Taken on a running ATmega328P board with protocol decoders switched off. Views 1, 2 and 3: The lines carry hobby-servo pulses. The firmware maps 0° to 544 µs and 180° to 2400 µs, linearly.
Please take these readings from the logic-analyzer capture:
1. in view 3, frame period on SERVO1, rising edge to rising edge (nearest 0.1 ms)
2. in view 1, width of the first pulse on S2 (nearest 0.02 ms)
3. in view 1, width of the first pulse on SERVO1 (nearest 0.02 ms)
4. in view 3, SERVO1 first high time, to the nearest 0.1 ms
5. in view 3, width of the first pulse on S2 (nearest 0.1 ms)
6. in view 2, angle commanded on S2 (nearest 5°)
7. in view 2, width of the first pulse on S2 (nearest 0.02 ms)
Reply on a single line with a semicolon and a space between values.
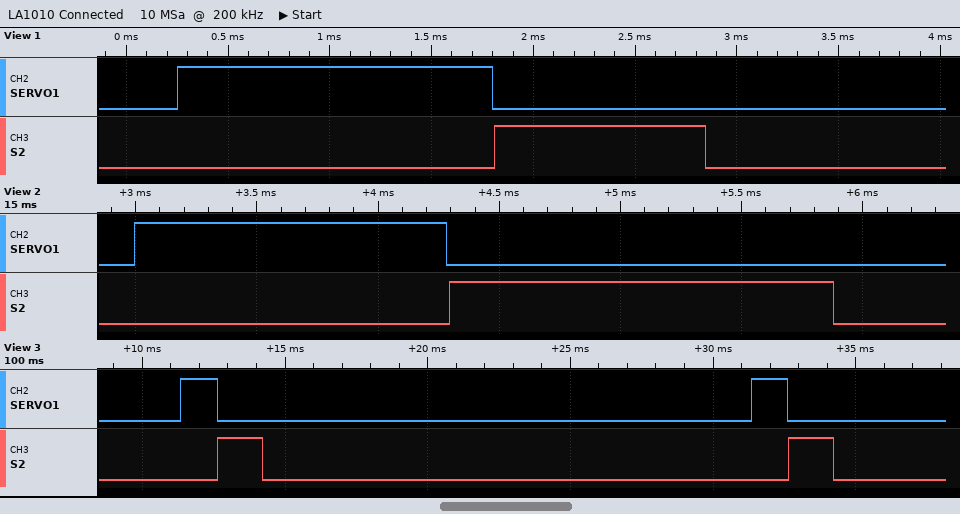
20.0 ms; 1.04 ms; 1.54 ms; 1.3 ms; 1.6 ms; 100°; 1.58 ms
